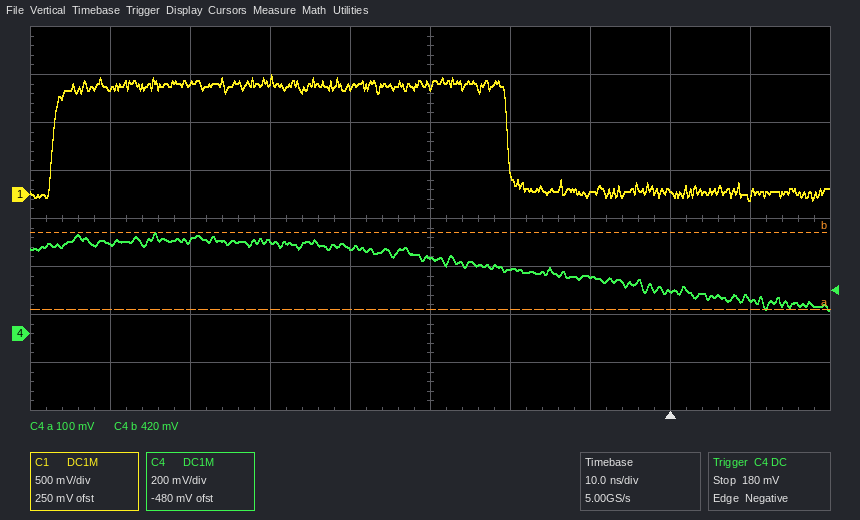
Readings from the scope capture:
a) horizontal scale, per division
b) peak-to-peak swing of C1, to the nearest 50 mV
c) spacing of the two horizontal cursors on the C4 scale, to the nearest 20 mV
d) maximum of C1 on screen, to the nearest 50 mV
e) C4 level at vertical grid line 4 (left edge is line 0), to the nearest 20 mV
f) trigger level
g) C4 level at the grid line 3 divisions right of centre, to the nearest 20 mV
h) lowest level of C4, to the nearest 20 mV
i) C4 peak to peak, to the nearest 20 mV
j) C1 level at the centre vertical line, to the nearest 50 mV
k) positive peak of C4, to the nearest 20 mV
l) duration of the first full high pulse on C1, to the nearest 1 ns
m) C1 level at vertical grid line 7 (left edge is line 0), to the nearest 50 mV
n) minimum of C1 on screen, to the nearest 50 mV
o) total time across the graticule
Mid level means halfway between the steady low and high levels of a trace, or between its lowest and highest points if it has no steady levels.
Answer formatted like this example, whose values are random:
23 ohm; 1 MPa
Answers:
10 ns; 1.30 V; 320 mV; 1.25 V; 360 mV; 180 mV; 180 mV; 100 mV; 320 mV; 1.15 V; 420 mV; 57 ns; 0 mV; -50 mV; 100 ns
